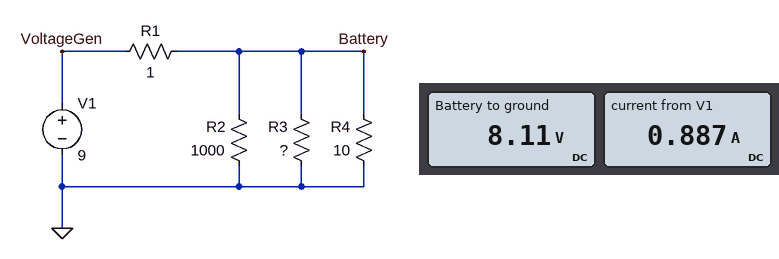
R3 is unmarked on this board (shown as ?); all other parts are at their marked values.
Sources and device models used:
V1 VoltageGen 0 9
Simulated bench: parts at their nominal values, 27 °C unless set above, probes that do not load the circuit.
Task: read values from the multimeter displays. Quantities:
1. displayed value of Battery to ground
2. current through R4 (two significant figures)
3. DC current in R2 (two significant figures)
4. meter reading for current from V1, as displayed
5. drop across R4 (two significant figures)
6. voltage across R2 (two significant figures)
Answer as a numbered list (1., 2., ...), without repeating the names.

1. 8.11 V
2. 810 mA
3. 8.1 mA
4. 0.887 A
5. 8.1 V
6. 8.1 V
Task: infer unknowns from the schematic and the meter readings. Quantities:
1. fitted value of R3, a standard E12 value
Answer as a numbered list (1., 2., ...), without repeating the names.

1. 120 Ω
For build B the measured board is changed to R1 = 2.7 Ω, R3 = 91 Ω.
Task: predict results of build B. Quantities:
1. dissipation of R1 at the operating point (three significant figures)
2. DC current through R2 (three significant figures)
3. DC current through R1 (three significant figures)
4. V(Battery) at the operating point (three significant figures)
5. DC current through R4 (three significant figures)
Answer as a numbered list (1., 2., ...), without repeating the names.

1. 1.62 W
2. 6.91 mA
3. 774 mA
4. 6.91 V
5. 691 mA
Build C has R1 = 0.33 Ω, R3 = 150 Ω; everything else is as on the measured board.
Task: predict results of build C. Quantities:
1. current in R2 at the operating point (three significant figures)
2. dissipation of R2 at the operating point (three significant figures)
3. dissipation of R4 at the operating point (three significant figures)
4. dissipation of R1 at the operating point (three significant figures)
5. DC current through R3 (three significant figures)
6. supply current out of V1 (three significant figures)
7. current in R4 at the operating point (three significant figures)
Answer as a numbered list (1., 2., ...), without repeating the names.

1. 8.69 mA
2. 75.5 mW
3. 7.55 W
4. 289 mW
5. 57.9 mA
6. 936 mA
7. 869 mA
